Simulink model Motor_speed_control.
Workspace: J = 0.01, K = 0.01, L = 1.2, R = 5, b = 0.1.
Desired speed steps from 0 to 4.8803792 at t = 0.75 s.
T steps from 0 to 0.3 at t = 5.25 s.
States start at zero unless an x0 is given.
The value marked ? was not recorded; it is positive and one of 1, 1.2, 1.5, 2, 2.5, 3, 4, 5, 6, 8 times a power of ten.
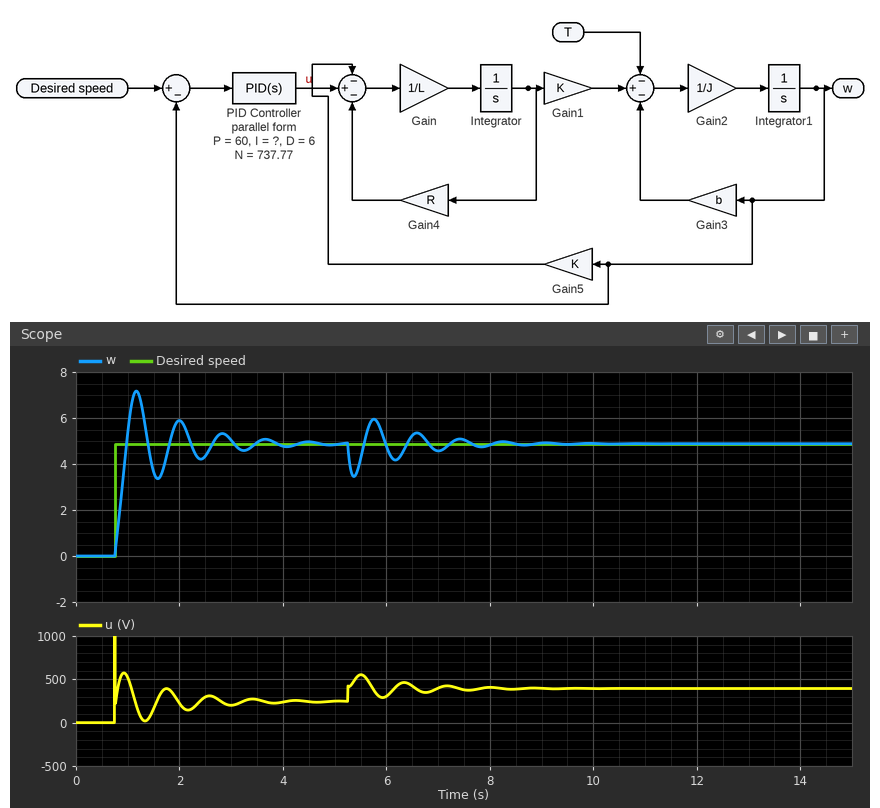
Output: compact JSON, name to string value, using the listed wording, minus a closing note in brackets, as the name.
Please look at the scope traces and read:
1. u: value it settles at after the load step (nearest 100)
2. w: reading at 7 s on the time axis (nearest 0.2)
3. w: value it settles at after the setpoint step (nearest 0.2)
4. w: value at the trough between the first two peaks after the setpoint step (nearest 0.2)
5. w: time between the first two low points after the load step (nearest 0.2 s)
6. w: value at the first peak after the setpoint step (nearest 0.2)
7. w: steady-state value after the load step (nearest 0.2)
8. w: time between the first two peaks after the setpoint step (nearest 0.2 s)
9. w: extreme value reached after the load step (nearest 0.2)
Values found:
{"u: value it settles at after the load step": "400", "w: reading at 7 s on the time axis": "4.6", "w: value it settles at after the setpoint step": "4.8", "w: value at the trough between the first two peaks after the setpoint step": "3.4", "w: time between the first two low points after the load step": "0.8 s", "w: value at the first peak after the setpoint step": "7.2", "w: steady-state value after the load step": "4.8", "w: time between the first two peaks after the setpoint step": "0.8 s", "w: extreme value reached after the load step": "3.4"}
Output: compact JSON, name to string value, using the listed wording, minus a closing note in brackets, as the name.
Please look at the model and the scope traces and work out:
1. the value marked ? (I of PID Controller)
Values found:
{"the value marked ?": "1200"}
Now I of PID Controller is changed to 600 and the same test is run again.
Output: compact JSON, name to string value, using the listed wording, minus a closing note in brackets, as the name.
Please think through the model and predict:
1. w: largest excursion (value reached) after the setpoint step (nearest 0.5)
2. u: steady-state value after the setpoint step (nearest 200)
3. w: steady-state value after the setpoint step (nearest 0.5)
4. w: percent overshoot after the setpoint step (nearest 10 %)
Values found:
{"w: largest excursion (value reached) after the setpoint step": "6.0", "u: steady-state value after the setpoint step": "200", "w: steady-state value after the setpoint step": "5.0", "w: percent overshoot after the setpoint step": "20 %"}
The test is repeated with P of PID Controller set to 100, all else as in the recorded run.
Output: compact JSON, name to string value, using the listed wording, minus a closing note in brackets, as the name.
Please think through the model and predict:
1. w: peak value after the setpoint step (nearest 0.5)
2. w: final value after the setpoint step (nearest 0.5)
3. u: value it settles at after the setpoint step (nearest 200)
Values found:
{"w: peak value after the setpoint step": "6.5", "w: final value after the setpoint step": "5.0", "u: value it settles at after the setpoint step": "200"}
